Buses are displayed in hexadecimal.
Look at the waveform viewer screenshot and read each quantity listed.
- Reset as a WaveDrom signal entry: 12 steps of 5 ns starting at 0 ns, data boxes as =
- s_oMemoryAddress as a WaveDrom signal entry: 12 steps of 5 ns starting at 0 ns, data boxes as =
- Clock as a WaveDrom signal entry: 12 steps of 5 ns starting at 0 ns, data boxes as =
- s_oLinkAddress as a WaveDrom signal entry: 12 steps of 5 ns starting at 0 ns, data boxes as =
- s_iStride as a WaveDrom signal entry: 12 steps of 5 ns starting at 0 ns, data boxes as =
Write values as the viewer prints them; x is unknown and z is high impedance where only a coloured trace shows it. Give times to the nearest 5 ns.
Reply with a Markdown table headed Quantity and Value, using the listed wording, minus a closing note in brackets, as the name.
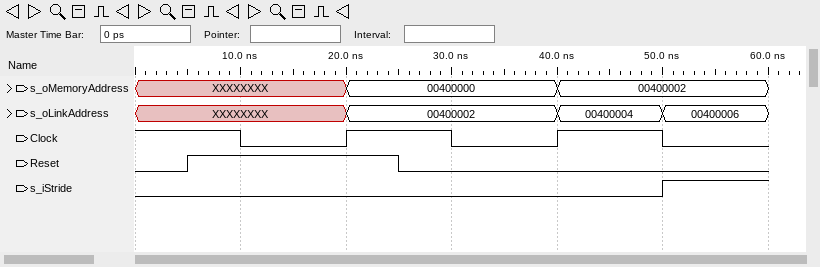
| Quantity | Value |
|---|---|
| Reset as a WaveDrom signal entry: 12 steps of 5 ns starting at 0 ns, data boxes as = | {name: 'Reset', wave: '01...0......'} |
| s_oMemoryAddress as a WaveDrom signal entry: 12 steps of 5 ns starting at 0 ns, data boxes as = | {name: 's_oMemoryAddress', wave: 'x...=...=...', data: '00400000 00400002'} |
| Clock as a WaveDrom signal entry: 12 steps of 5 ns starting at 0 ns, data boxes as = | {name: 'Clock', wave: '1.0.1.0.1.0.'} |
| s_oLinkAddress as a WaveDrom signal entry: 12 steps of 5 ns starting at 0 ns, data boxes as = | {name: 's_oLinkAddress', wave: 'x...=...=.=.', data: '00400002 00400004 00400006'} |
| s_iStride as a WaveDrom signal entry: 12 steps of 5 ns starting at 0 ns, data boxes as = | {name: 's_iStride', wave: '0.........1.'} |
